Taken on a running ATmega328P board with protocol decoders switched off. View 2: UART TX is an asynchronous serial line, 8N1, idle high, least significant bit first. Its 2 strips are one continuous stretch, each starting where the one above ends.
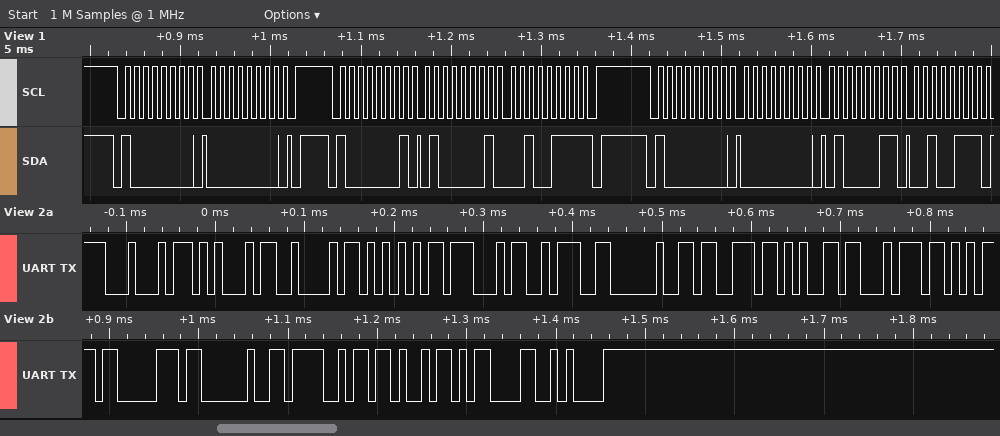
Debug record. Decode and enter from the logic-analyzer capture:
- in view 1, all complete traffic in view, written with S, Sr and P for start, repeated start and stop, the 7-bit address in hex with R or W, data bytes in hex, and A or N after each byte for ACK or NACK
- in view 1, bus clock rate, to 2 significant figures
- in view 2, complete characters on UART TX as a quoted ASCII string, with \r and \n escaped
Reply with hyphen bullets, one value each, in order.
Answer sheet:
- S 40W A 00 A P S 40R A 41 A 27 N P S 40W A 00 A 43 A 27 A
- 100 kHz
- "DEBUG: setup OK\r\n"
